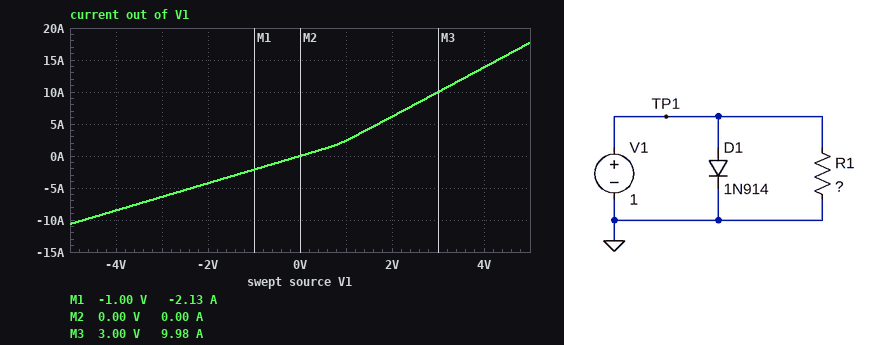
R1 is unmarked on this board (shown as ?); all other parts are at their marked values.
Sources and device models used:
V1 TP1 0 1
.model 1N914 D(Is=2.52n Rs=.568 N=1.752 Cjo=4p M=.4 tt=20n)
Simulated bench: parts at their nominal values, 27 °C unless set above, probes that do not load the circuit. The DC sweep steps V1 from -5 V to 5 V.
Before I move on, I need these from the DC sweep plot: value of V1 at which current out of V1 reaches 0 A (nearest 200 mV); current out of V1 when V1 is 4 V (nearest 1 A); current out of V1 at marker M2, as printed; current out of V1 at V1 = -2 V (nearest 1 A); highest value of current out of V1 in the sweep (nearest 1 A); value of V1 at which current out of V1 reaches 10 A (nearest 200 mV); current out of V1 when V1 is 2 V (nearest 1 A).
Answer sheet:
0 V
14 A
0.00 A
-4 A
18 A
3.0 V
6 A
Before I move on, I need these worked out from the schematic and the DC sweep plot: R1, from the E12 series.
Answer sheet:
0.47 Ω
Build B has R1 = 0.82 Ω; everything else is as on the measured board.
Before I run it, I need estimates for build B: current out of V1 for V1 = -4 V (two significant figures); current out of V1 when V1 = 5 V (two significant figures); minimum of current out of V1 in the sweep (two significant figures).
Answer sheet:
-4.9 A
13 A
-6.1 A
